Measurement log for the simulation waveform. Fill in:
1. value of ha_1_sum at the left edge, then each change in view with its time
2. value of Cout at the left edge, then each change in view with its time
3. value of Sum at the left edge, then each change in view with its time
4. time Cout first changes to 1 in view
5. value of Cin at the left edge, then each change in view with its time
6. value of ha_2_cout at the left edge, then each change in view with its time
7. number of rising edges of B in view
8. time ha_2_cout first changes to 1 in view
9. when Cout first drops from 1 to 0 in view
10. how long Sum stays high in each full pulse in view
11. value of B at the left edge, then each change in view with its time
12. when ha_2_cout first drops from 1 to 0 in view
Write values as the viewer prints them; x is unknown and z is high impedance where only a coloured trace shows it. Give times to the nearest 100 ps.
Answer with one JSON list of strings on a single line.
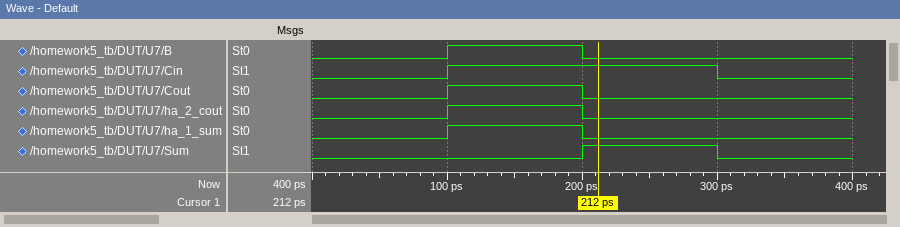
["0, 1 at 100 ps, 0 at 200 ps", "0, 1 at 100 ps, 0 at 200 ps", "0, 1 at 200 ps, 0 at 300 ps", "100 ps", "0, 1 at 100 ps, 0 at 300 ps", "0, 1 at 100 ps, 0 at 200 ps", "1", "100 ps", "200 ps", "100 ps", "0, 1 at 100 ps, 0 at 200 ps", "200 ps"]
